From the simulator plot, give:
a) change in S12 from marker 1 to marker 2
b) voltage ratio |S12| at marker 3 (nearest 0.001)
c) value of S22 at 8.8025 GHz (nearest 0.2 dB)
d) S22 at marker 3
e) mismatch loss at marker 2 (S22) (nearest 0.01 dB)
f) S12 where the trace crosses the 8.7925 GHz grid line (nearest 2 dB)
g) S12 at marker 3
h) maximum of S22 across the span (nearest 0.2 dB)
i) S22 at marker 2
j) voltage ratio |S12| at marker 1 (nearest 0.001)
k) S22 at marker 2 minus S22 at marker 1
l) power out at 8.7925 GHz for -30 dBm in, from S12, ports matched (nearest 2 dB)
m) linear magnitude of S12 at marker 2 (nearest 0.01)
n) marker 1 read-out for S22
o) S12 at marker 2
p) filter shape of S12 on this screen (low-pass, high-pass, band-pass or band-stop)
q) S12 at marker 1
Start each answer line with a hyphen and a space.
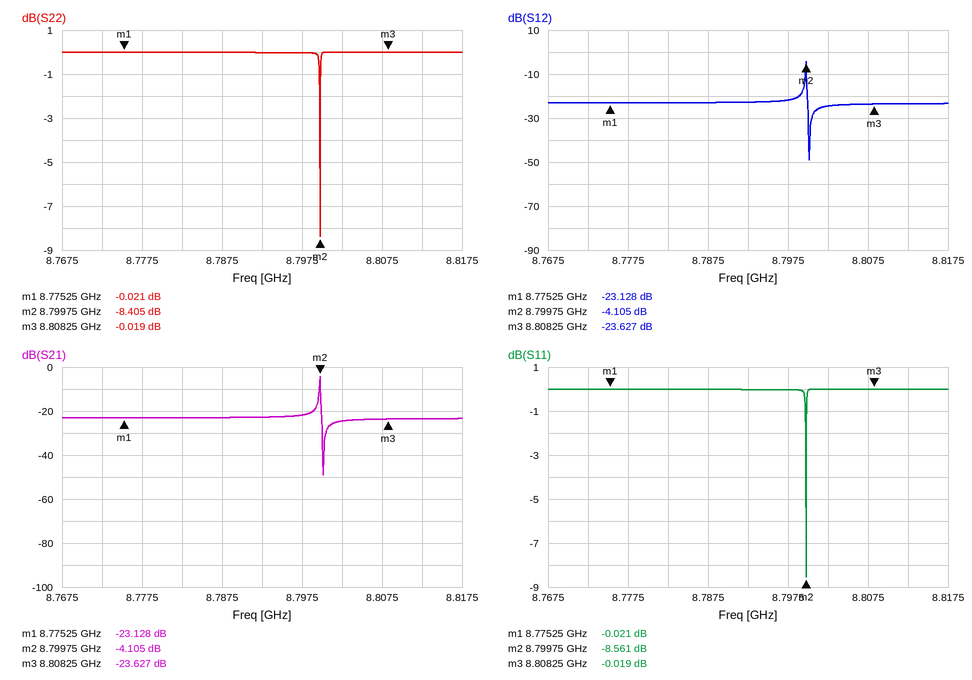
- 19.023 dB
- 0.066
- 0.0 dB
- -0.019 dB
- 0.68 dB
- -22 dB
- -23.627 dB
- 0.0 dB
- -8.405 dB
- 0.070
- -8.384 dB
- -52 dBm
- 0.62
- -0.021 dB
- -4.105 dB
- band-pass
- -23.128 dB
